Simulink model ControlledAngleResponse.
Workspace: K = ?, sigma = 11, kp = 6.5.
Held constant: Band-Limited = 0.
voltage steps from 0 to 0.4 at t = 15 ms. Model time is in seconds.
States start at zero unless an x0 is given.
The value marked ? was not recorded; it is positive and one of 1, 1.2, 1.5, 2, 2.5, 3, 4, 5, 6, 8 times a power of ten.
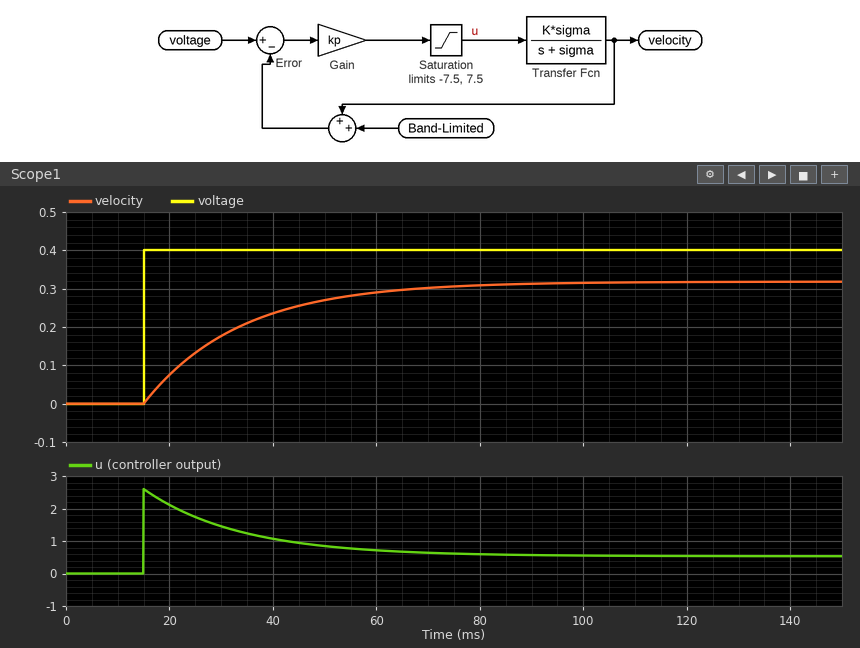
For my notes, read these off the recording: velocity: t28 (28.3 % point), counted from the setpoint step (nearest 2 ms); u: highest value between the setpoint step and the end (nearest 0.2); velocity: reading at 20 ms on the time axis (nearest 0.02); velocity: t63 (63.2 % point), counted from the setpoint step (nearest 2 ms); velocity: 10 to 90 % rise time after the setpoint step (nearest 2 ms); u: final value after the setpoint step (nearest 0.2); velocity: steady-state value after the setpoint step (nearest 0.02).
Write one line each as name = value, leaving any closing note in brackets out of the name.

velocity: t28 (28.3 % point), counted from the setpoint step = 6 ms
u: highest value between the setpoint step and the end = 2.6
velocity: reading at 20 ms on the time axis = 0.08
velocity: t63 (63.2 % point), counted from the setpoint step = 18 ms
velocity: 10 to 90 % rise time after the setpoint step = 40 ms
u: final value after the setpoint step = 0.6
velocity: steady-state value after the setpoint step = 0.32
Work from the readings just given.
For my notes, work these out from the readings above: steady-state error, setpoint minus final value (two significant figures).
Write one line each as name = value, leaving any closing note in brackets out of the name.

steady-state error, setpoint minus final value = 0.080
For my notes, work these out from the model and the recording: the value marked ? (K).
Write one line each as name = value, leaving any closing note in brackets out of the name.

the value marked ? = 0.6
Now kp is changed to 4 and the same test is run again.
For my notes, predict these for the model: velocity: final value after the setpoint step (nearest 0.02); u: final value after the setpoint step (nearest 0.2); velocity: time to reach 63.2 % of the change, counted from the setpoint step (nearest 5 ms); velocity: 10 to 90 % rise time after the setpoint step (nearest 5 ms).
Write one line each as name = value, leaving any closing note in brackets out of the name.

velocity: final value after the setpoint step = 0.28
u: final value after the setpoint step = 0.4
velocity: time to reach 63.2 % of the change, counted from the setpoint step = 25 ms
velocity: 10 to 90 % rise time after the setpoint step = 60 ms
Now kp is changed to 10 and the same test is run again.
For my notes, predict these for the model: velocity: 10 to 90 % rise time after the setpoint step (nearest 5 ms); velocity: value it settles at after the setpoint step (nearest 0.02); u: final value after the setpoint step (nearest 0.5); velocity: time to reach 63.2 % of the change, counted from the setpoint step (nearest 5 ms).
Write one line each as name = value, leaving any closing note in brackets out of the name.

velocity: 10 to 90 % rise time after the setpoint step = 30 ms
velocity: value it settles at after the setpoint step = 0.34
u: final value after the setpoint step = 0.5
velocity: time to reach 63.2 % of the change, counted from the setpoint step = 15 ms
